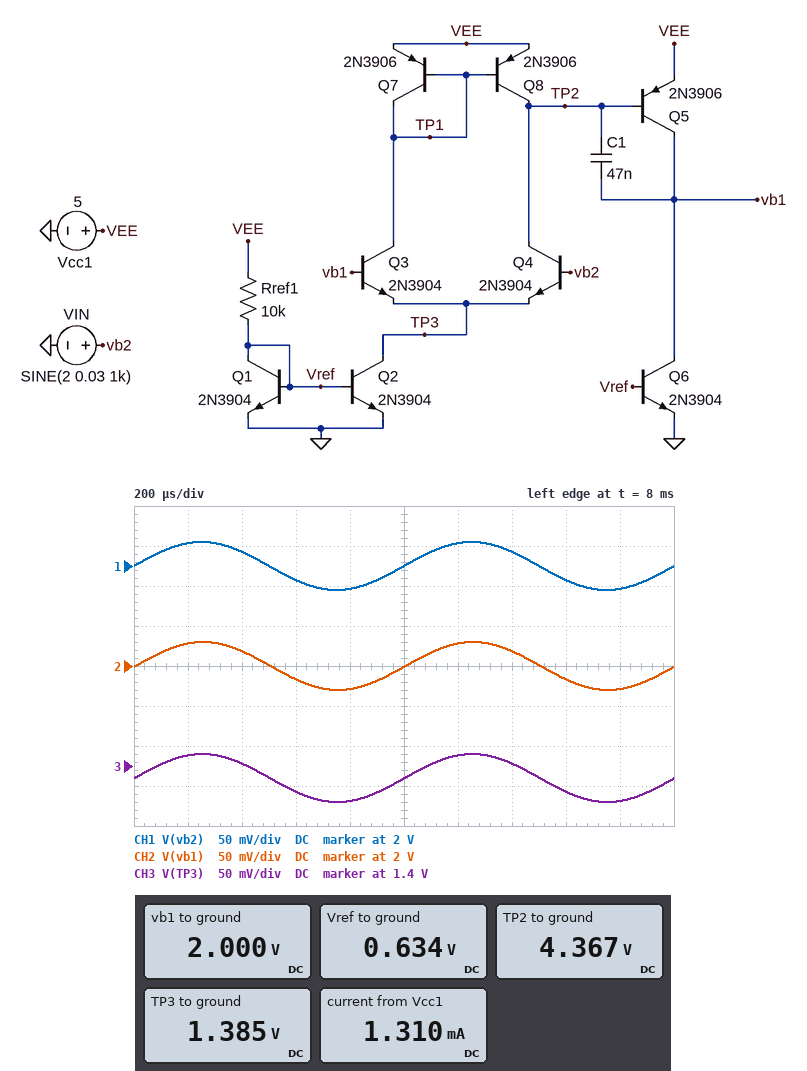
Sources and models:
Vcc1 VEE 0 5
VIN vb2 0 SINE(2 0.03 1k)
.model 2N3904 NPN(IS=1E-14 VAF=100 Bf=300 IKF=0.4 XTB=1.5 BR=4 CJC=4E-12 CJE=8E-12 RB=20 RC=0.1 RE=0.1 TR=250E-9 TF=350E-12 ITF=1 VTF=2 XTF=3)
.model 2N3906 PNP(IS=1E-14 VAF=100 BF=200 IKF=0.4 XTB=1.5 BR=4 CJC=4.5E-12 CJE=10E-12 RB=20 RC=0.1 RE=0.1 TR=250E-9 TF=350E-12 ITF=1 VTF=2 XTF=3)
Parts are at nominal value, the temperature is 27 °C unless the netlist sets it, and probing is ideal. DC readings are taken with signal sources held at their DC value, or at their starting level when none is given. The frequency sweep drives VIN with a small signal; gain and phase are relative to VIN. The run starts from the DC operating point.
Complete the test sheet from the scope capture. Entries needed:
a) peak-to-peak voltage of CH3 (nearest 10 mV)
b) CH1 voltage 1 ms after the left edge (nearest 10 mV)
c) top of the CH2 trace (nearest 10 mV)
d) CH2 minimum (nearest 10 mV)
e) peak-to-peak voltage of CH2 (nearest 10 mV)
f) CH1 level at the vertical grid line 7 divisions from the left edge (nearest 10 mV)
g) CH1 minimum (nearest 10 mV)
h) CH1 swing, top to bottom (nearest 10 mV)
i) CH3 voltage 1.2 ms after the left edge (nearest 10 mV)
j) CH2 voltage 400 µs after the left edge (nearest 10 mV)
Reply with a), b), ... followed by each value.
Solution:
a) 60 mV
b) 2.00 V
c) 2.03 V
d) 1.97 V
e) 60 mV
f) 2.02 V
g) 1.97 V
h) 60 mV
i) 1.41 V
j) 2.02 V
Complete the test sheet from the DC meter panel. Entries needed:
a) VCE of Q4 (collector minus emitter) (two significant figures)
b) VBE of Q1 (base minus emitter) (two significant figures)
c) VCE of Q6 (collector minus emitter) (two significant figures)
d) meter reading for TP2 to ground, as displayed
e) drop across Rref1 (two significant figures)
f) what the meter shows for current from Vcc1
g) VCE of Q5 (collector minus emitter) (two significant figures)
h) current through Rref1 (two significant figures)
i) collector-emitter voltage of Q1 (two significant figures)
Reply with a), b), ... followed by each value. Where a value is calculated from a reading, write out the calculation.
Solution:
a) 4.367 V - 1.385 V = 3.0 V
b) 634 mV = 630 mV
c) 2 V = 2.0 V
d) 4.367 V
e) 5 V - 634 mV = 4.4 V
f) 1.310 mA
g) 2 V - 5 V = -3.0 V
h) (5 V - 634 mV) / 10 kΩ = 440 µA
i) 634 mV = 630 mV
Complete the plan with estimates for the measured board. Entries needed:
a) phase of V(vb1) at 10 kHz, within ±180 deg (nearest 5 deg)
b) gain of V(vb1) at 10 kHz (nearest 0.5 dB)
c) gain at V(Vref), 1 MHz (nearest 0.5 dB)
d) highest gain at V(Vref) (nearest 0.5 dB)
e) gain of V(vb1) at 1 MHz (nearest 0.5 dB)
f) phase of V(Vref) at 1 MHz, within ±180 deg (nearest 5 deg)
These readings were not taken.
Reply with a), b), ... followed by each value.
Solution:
a) -20 deg
b) 0 dB
c) -60.0 dB
d) -28.0 dB
e) -0.5 dB
f) -90 deg
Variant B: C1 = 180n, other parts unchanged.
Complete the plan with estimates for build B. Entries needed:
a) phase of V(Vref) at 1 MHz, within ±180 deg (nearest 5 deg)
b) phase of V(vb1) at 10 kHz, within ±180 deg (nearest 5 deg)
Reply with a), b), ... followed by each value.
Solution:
a) -95 deg
b) -70 deg
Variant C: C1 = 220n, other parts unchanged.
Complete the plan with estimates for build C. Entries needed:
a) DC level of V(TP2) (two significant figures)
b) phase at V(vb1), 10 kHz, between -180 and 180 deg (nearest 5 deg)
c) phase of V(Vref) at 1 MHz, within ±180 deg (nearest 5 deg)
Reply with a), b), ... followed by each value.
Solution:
a) 4.4 V
b) -80 deg
c) -95 deg
